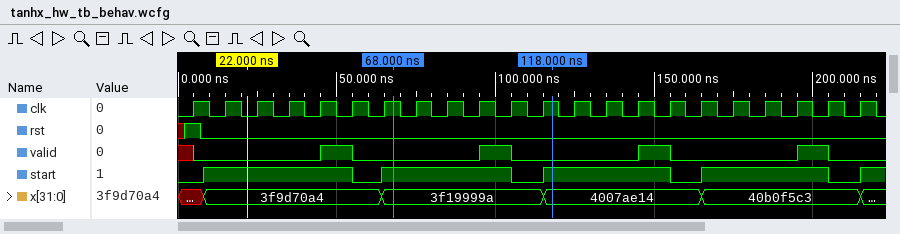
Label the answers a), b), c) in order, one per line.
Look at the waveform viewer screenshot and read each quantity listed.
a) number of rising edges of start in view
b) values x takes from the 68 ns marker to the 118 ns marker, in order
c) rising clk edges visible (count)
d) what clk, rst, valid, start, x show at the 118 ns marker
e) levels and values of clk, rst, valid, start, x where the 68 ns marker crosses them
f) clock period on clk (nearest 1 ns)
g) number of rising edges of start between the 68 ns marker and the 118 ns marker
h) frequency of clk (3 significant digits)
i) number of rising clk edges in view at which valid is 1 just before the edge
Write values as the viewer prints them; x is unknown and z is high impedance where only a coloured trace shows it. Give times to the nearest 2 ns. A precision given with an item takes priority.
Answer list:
a) 5
b) 3f19999a, 4007ae14
c) 22
d) clk=1, rst=0, valid=0, start=1, x=4007ae14
e) clk=1, rst=0, valid=0, start=1, x=3f19999a
f) 10 ns
g) 1
h) 100 MHz
i) 4
